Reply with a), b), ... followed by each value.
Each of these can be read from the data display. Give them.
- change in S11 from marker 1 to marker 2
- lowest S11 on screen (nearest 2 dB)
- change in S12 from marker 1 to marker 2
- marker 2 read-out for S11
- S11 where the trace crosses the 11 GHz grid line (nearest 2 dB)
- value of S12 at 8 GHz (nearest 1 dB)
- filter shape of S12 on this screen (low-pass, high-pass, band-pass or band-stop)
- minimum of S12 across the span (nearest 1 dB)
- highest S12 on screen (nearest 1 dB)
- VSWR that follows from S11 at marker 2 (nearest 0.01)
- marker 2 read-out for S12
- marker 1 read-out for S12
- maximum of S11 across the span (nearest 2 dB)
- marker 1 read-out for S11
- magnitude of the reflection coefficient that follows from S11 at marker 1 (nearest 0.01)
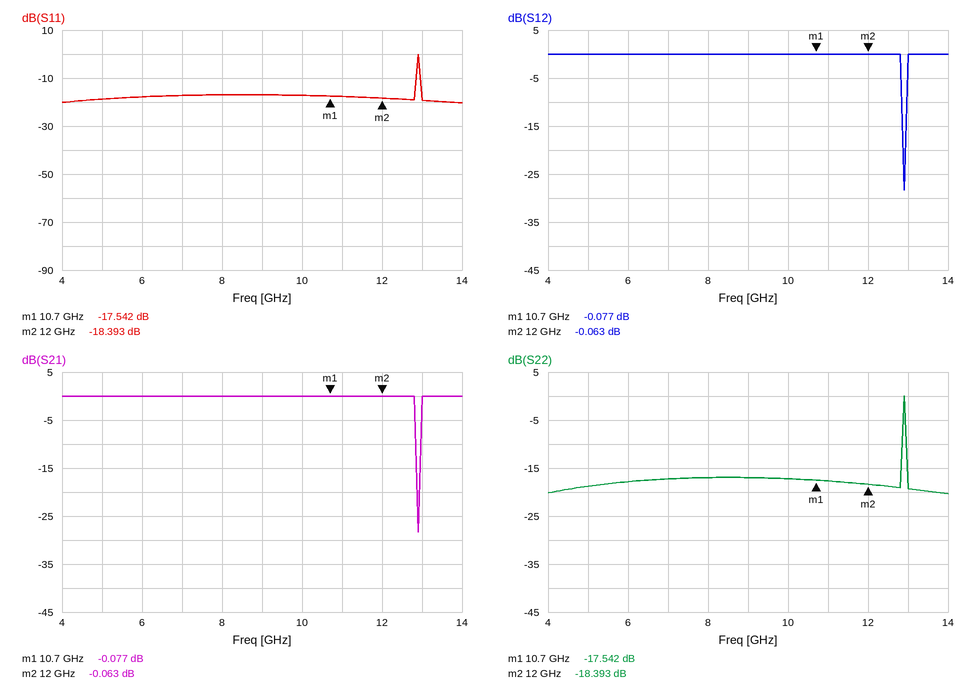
a) -0.851 dB
b) -20 dB
c) 0.014 dB
d) -18.393 dB
e) -18 dB
f) 0 dB
g) band-stop
h) -28 dB
i) 0 dB
j) 1.27
k) -0.063 dB
l) -0.077 dB
m) 0 dB
n) -17.542 dB
o) 0.13
